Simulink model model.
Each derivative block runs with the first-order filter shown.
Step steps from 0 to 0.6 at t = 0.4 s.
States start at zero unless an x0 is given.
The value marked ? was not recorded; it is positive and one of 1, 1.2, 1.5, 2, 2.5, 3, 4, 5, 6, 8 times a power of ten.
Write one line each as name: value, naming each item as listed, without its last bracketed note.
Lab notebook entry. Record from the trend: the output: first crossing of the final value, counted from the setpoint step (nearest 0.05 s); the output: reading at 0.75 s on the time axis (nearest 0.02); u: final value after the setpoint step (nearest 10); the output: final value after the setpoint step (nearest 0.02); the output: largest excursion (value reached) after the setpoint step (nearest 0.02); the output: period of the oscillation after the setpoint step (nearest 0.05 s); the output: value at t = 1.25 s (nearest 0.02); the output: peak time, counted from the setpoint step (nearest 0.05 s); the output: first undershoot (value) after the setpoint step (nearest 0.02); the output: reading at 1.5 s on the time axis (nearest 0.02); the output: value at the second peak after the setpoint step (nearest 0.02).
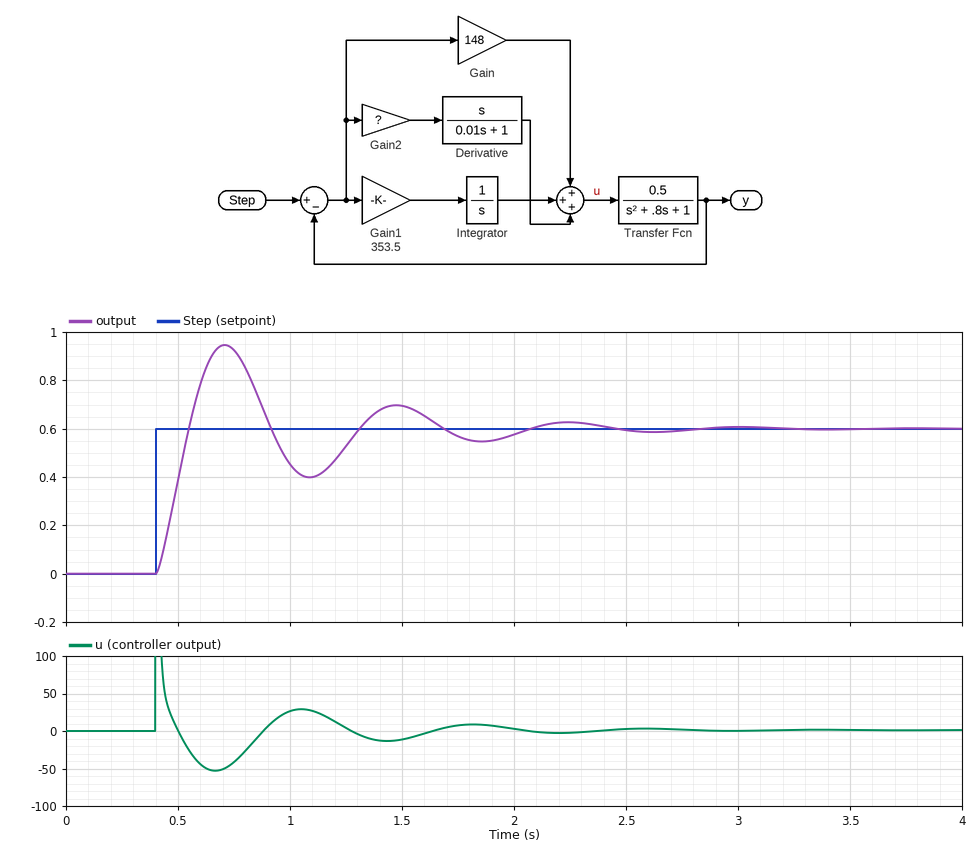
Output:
the output: first crossing of the final value, counted from the setpoint step: 0.15 s
the output: reading at 0.75 s on the time axis: 0.92
u: final value after the setpoint step: 0
the output: final value after the setpoint step: 0.60
the output: largest excursion (value reached) after the setpoint step: 0.94
the output: period of the oscillation after the setpoint step: 0.75 s
the output: value at t = 1.25 s: 0.52
the output: peak time, counted from the setpoint step: 0.30 s
the output: first undershoot (value) after the setpoint step: 0.40
the output: reading at 1.5 s on the time axis: 0.70
the output: value at the second peak after the setpoint step: 0.70
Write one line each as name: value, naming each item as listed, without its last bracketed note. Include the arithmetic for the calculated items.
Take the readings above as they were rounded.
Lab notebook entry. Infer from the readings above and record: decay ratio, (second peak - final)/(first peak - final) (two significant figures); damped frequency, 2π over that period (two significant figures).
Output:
decay ratio, (second peak - final)/(first peak - final): (0.7 - 0.6) / (0.94 - 0.6) = 0.29
damped frequency, 2π over that period: 2π / 0.75 = 8.4 rad/s
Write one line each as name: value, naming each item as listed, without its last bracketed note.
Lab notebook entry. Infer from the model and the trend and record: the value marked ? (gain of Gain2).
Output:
the value marked ?: 10
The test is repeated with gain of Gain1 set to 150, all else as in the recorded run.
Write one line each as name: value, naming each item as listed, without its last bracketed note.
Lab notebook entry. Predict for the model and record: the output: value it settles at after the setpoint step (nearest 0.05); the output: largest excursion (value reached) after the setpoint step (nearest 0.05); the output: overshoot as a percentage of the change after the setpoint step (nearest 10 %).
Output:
the output: value it settles at after the setpoint step: 0.60
the output: largest excursion (value reached) after the setpoint step: 0.90
the output: overshoot as a percentage of the change after the setpoint step: 50 %
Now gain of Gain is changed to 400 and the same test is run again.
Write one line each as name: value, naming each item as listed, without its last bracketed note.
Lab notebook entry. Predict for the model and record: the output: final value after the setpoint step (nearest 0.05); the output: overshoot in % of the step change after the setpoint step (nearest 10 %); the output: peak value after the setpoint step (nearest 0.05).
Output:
the output: final value after the setpoint step: 0.60
the output: overshoot in % of the step change after the setpoint step: 60 %
the output: peak value after the setpoint step: 1.00
